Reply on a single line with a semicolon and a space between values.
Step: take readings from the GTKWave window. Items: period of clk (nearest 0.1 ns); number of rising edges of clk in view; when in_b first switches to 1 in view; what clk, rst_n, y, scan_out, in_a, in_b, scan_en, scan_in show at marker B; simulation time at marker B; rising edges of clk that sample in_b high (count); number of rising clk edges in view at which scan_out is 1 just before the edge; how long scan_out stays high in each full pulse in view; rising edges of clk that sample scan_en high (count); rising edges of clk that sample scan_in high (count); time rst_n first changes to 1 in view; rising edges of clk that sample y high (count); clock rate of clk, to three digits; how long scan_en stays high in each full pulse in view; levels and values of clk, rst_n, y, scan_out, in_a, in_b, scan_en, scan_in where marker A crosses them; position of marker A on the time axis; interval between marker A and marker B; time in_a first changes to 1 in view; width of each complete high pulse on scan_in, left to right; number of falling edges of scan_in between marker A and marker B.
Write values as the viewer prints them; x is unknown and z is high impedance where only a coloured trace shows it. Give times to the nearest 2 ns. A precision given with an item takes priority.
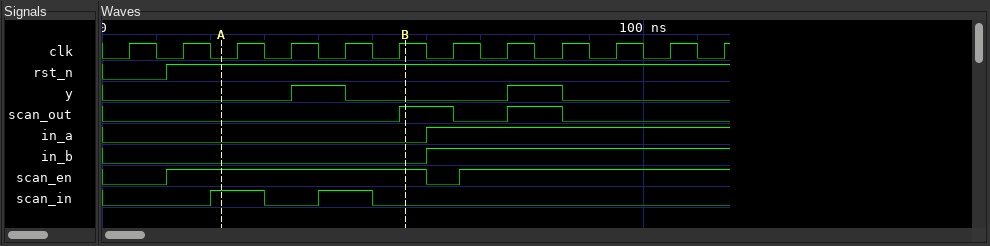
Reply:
10 ns; 12; 60 ns; clk=1, rst_n=1, y=0, scan_out=1, in_a=0, in_b=0, scan_en=1, scan_in=0; 56 ns; 6; 2; 10 ns, 10 ns; 10; 2; 12 ns; 2; 100 MHz; 48 ns; clk=0, rst_n=1, y=0, scan_out=0, in_a=0, in_b=0, scan_en=1, scan_in=1; 22 ns; 34 ns; 60 ns; 10 ns, 10 ns; 2
